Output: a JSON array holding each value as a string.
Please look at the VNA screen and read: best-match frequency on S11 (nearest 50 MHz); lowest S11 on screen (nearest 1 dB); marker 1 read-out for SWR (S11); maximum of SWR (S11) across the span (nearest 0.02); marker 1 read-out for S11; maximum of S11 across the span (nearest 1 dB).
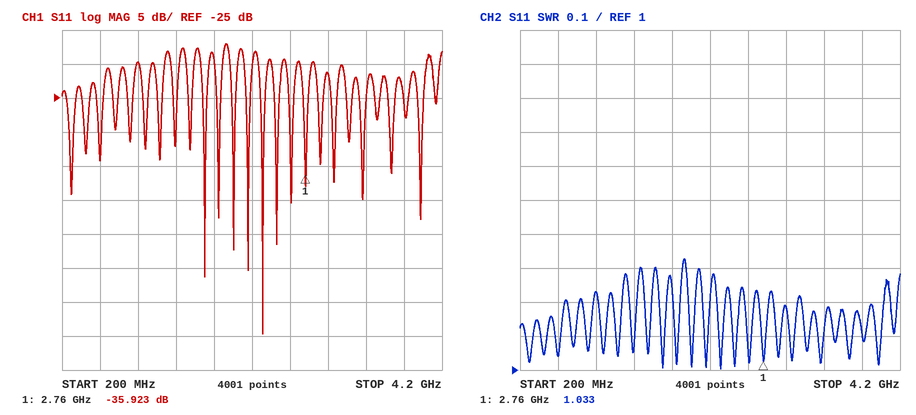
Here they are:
["2.30 GHz", "-60 dB", "1.033", "1.32", "-35.923 dB", "-17 dB"]
